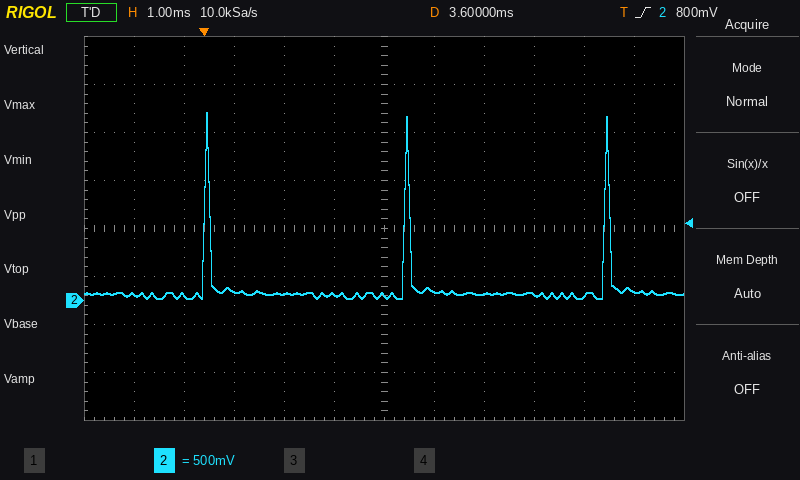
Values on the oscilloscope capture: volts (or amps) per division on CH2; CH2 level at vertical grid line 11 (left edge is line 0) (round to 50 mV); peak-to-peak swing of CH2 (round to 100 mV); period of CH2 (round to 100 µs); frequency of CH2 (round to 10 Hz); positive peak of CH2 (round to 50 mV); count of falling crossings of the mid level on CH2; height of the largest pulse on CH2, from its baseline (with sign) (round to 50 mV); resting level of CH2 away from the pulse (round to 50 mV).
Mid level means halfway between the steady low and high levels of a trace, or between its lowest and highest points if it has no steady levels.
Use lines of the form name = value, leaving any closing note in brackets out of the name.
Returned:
volts (or amps) per division on CH2 = 500 mV
CH2 level at vertical grid line 11 (left edge is line 0) = 100 mV
peak-to-peak swing of CH2 = 1.90 V
period of CH2 = 4.0 ms
frequency of CH2 = 250 Hz
positive peak of CH2 = 1.95 V
count of falling crossings of the mid level on CH2 = 3
height of the largest pulse on CH2, from its baseline (with sign) = +1.90 V
resting level of CH2 away from the pulse = 50 mV
